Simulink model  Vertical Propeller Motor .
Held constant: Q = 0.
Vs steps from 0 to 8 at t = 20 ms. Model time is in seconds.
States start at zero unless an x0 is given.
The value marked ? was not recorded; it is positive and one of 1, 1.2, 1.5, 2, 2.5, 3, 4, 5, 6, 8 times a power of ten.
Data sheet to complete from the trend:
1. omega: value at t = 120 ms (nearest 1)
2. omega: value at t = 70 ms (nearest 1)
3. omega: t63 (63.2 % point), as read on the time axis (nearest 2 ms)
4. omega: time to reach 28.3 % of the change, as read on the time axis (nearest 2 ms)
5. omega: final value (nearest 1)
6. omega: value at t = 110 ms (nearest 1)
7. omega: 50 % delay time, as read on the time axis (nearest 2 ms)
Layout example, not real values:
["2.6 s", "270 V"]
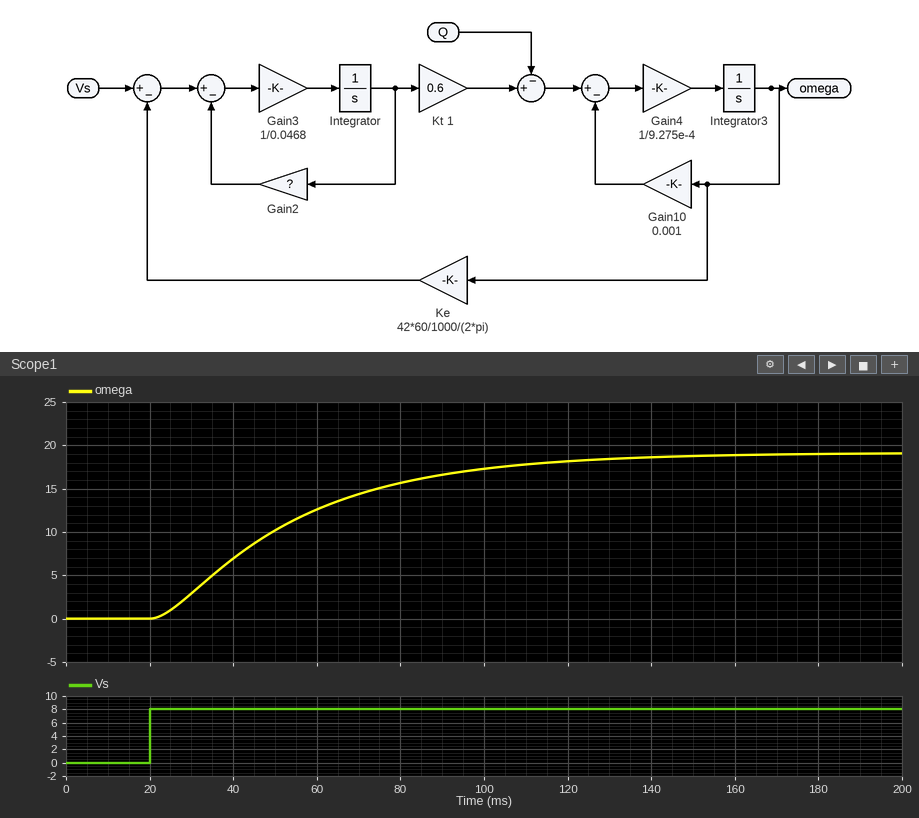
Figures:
["18", "14", "58 ms", "36 ms", "19", "18", "48 ms"]
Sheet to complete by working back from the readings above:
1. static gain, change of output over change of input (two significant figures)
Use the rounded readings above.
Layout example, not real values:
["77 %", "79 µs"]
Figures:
["2.4"]
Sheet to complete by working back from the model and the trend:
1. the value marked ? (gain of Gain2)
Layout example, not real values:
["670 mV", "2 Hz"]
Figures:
["10"]
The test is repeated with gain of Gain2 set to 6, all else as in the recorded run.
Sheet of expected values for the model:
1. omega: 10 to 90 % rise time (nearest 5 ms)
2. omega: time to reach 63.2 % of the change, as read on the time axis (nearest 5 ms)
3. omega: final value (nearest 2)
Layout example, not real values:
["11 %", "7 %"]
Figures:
["35 ms", "45 ms", "20"]
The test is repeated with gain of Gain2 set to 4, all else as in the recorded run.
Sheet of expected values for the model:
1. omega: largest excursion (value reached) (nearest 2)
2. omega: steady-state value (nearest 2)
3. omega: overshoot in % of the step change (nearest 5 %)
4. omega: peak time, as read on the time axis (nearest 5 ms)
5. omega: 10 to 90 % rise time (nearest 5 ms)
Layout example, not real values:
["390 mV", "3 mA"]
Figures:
["22", "20", "10 %", "70 ms", "25 ms"]
